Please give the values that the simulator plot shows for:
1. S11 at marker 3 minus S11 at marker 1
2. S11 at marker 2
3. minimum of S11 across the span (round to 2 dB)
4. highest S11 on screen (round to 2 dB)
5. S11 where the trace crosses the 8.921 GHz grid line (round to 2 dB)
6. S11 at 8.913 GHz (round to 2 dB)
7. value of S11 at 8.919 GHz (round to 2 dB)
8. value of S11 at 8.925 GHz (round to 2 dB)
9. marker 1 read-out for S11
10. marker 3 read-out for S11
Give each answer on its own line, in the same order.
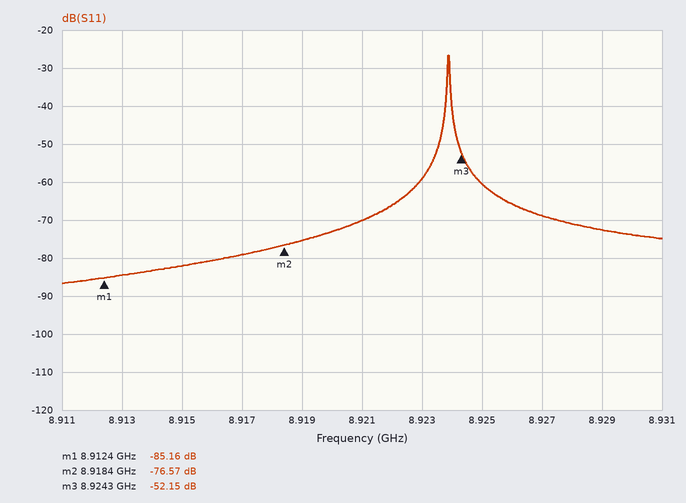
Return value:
33.01 dB
-76.57 dB
-86 dB
-26 dB
-70 dB
-84 dB
-76 dB
-60 dB
-85.16 dB
-52.15 dB
